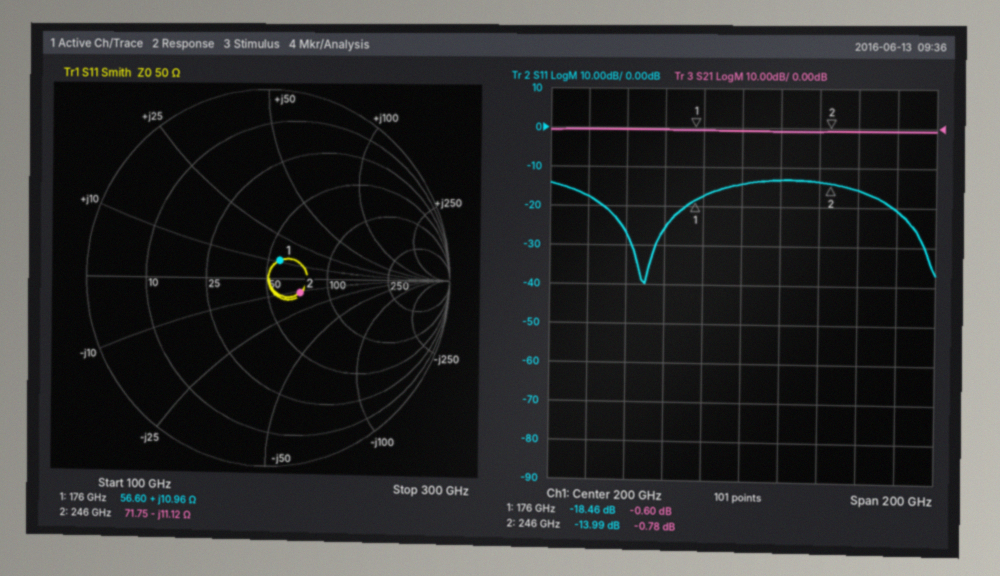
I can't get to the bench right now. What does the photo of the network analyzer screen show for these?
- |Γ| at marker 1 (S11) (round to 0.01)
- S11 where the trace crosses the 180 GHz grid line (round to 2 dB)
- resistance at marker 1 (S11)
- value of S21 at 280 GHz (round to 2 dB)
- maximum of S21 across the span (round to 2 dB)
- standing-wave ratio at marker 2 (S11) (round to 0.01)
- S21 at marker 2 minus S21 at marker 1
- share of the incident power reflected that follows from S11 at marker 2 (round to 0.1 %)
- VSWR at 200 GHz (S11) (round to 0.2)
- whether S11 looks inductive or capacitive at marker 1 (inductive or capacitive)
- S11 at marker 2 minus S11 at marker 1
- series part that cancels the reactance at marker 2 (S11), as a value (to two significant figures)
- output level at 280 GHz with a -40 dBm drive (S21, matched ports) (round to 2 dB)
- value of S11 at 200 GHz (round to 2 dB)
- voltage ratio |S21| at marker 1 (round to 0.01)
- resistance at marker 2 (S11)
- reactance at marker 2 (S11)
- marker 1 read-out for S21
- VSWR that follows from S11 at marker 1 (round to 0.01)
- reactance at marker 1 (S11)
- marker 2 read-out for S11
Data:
0.12
-18 dB
56.60 Ω
0 dB
0 dB
1.50
-0.18 dB
4.0 %
1.4
inductive
4.47 dB
7.2 pH
-40 dBm
-14 dB
0.93
71.75 Ω
-11.12 Ω
-0.60 dB
1.27
+10.96 Ω
-13.99 dB
